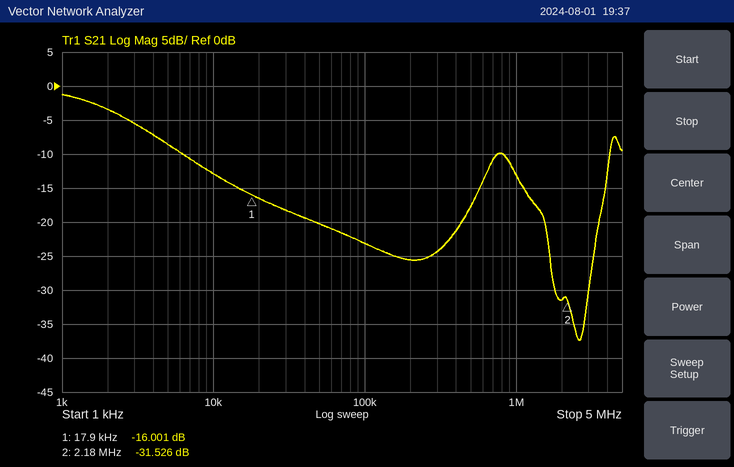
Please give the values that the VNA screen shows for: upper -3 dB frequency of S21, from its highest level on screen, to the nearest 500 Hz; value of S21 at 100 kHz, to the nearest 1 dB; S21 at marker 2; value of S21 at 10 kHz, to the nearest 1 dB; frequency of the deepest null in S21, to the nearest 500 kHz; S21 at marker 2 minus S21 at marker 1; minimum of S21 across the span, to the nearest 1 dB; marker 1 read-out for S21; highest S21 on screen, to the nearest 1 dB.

2.5 kHz
-23 dB
-31.526 dB
-13 dB
2.5 MHz
-15.525 dB
-37 dB
-16.001 dB
-1 dB
